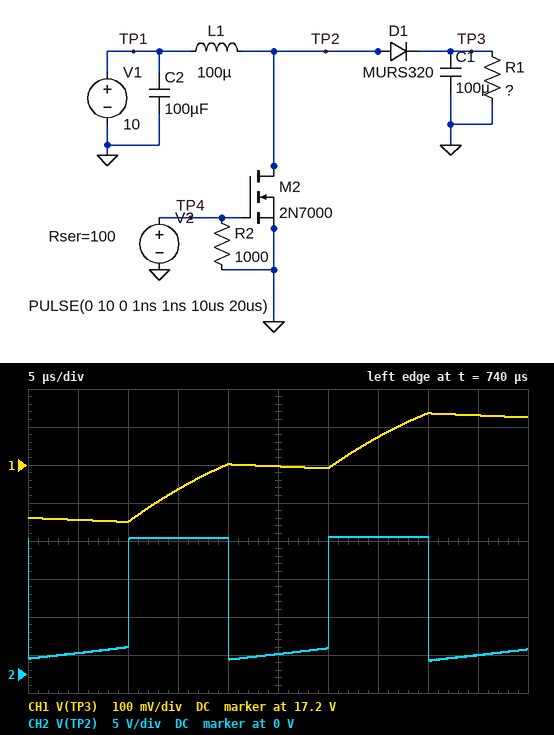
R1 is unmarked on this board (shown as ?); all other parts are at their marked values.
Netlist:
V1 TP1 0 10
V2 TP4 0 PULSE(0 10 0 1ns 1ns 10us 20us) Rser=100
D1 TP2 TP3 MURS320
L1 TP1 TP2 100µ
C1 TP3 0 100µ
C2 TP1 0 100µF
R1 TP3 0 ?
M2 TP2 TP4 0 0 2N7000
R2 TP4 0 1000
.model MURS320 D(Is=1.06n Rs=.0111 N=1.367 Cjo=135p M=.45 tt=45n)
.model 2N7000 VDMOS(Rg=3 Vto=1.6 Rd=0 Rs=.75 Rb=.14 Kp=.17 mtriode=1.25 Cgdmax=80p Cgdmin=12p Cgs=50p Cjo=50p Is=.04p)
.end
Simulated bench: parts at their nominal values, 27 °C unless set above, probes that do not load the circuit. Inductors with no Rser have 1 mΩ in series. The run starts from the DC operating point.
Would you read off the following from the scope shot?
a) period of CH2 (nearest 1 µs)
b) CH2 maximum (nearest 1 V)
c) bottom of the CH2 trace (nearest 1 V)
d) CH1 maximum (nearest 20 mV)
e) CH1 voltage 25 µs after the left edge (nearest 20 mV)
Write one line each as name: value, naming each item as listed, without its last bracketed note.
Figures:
period of CH2: 20 µs
CH2 maximum: 18 V
bottom of the CH2 trace: 2 V
CH1 maximum: 17.34 V
CH1 voltage 25 µs after the left edge: 17.20 V
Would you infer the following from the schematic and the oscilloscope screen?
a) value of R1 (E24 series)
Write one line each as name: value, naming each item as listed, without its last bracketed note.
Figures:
value of R1: 160 Ω
